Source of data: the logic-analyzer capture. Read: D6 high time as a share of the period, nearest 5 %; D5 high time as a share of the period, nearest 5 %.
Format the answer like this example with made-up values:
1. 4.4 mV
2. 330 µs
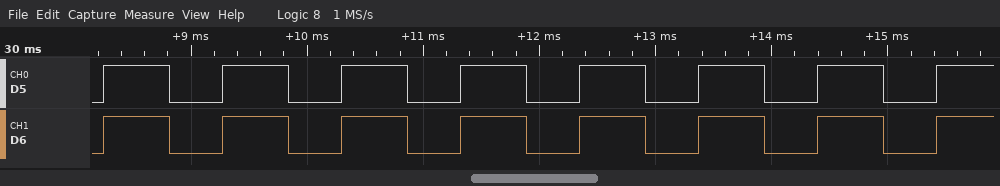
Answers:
1. 55 %
2. 55 %
